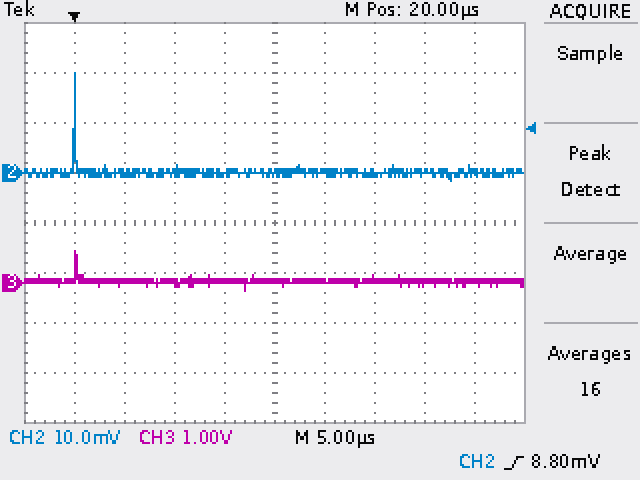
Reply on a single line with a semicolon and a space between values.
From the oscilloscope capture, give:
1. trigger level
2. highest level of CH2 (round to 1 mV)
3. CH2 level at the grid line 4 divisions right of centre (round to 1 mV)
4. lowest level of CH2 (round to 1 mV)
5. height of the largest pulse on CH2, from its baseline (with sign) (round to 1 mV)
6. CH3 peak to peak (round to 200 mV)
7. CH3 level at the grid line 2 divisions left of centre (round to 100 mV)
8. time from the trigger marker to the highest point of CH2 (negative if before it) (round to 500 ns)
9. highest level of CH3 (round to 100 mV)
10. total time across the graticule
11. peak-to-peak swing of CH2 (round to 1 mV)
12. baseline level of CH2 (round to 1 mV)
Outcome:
8.80 mV; 20 mV; 0 mV; -2 mV; +20 mV; 800 mV; 0.0 V; 0.0 µs; 600 mV; 50 µs; 22 mV; 0 mV
